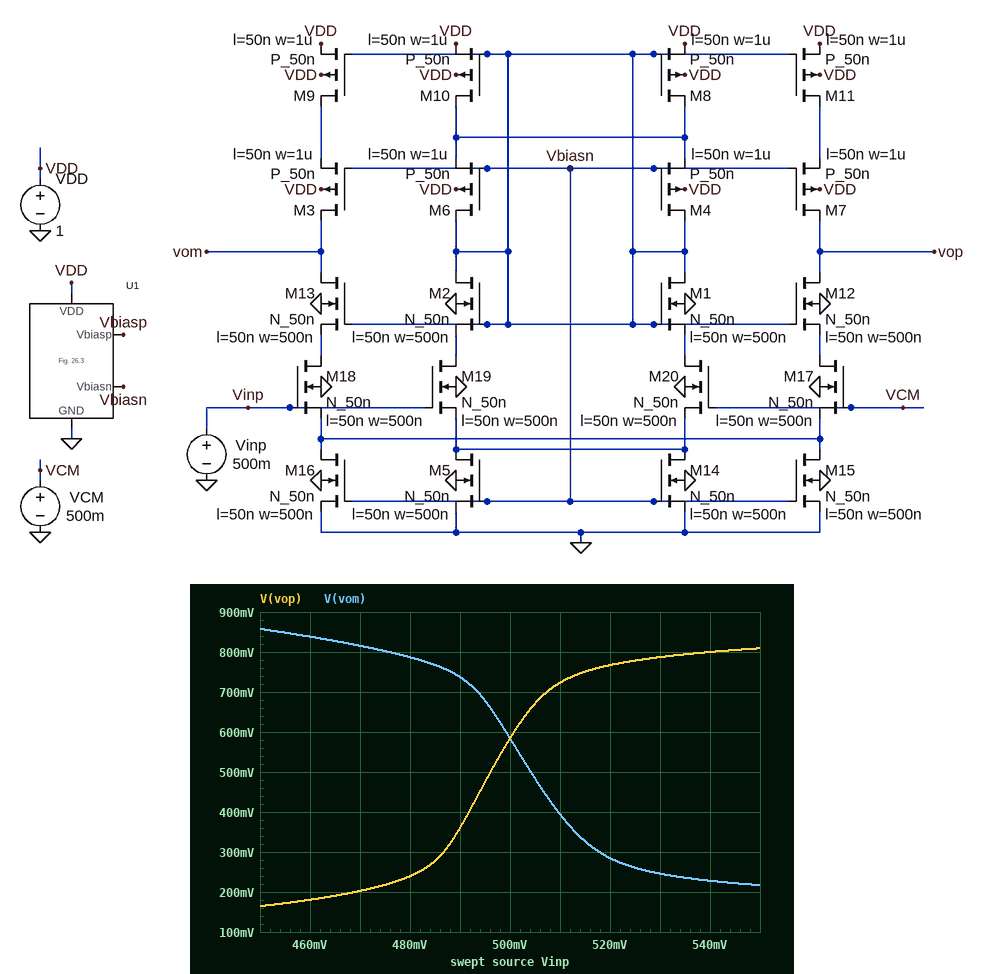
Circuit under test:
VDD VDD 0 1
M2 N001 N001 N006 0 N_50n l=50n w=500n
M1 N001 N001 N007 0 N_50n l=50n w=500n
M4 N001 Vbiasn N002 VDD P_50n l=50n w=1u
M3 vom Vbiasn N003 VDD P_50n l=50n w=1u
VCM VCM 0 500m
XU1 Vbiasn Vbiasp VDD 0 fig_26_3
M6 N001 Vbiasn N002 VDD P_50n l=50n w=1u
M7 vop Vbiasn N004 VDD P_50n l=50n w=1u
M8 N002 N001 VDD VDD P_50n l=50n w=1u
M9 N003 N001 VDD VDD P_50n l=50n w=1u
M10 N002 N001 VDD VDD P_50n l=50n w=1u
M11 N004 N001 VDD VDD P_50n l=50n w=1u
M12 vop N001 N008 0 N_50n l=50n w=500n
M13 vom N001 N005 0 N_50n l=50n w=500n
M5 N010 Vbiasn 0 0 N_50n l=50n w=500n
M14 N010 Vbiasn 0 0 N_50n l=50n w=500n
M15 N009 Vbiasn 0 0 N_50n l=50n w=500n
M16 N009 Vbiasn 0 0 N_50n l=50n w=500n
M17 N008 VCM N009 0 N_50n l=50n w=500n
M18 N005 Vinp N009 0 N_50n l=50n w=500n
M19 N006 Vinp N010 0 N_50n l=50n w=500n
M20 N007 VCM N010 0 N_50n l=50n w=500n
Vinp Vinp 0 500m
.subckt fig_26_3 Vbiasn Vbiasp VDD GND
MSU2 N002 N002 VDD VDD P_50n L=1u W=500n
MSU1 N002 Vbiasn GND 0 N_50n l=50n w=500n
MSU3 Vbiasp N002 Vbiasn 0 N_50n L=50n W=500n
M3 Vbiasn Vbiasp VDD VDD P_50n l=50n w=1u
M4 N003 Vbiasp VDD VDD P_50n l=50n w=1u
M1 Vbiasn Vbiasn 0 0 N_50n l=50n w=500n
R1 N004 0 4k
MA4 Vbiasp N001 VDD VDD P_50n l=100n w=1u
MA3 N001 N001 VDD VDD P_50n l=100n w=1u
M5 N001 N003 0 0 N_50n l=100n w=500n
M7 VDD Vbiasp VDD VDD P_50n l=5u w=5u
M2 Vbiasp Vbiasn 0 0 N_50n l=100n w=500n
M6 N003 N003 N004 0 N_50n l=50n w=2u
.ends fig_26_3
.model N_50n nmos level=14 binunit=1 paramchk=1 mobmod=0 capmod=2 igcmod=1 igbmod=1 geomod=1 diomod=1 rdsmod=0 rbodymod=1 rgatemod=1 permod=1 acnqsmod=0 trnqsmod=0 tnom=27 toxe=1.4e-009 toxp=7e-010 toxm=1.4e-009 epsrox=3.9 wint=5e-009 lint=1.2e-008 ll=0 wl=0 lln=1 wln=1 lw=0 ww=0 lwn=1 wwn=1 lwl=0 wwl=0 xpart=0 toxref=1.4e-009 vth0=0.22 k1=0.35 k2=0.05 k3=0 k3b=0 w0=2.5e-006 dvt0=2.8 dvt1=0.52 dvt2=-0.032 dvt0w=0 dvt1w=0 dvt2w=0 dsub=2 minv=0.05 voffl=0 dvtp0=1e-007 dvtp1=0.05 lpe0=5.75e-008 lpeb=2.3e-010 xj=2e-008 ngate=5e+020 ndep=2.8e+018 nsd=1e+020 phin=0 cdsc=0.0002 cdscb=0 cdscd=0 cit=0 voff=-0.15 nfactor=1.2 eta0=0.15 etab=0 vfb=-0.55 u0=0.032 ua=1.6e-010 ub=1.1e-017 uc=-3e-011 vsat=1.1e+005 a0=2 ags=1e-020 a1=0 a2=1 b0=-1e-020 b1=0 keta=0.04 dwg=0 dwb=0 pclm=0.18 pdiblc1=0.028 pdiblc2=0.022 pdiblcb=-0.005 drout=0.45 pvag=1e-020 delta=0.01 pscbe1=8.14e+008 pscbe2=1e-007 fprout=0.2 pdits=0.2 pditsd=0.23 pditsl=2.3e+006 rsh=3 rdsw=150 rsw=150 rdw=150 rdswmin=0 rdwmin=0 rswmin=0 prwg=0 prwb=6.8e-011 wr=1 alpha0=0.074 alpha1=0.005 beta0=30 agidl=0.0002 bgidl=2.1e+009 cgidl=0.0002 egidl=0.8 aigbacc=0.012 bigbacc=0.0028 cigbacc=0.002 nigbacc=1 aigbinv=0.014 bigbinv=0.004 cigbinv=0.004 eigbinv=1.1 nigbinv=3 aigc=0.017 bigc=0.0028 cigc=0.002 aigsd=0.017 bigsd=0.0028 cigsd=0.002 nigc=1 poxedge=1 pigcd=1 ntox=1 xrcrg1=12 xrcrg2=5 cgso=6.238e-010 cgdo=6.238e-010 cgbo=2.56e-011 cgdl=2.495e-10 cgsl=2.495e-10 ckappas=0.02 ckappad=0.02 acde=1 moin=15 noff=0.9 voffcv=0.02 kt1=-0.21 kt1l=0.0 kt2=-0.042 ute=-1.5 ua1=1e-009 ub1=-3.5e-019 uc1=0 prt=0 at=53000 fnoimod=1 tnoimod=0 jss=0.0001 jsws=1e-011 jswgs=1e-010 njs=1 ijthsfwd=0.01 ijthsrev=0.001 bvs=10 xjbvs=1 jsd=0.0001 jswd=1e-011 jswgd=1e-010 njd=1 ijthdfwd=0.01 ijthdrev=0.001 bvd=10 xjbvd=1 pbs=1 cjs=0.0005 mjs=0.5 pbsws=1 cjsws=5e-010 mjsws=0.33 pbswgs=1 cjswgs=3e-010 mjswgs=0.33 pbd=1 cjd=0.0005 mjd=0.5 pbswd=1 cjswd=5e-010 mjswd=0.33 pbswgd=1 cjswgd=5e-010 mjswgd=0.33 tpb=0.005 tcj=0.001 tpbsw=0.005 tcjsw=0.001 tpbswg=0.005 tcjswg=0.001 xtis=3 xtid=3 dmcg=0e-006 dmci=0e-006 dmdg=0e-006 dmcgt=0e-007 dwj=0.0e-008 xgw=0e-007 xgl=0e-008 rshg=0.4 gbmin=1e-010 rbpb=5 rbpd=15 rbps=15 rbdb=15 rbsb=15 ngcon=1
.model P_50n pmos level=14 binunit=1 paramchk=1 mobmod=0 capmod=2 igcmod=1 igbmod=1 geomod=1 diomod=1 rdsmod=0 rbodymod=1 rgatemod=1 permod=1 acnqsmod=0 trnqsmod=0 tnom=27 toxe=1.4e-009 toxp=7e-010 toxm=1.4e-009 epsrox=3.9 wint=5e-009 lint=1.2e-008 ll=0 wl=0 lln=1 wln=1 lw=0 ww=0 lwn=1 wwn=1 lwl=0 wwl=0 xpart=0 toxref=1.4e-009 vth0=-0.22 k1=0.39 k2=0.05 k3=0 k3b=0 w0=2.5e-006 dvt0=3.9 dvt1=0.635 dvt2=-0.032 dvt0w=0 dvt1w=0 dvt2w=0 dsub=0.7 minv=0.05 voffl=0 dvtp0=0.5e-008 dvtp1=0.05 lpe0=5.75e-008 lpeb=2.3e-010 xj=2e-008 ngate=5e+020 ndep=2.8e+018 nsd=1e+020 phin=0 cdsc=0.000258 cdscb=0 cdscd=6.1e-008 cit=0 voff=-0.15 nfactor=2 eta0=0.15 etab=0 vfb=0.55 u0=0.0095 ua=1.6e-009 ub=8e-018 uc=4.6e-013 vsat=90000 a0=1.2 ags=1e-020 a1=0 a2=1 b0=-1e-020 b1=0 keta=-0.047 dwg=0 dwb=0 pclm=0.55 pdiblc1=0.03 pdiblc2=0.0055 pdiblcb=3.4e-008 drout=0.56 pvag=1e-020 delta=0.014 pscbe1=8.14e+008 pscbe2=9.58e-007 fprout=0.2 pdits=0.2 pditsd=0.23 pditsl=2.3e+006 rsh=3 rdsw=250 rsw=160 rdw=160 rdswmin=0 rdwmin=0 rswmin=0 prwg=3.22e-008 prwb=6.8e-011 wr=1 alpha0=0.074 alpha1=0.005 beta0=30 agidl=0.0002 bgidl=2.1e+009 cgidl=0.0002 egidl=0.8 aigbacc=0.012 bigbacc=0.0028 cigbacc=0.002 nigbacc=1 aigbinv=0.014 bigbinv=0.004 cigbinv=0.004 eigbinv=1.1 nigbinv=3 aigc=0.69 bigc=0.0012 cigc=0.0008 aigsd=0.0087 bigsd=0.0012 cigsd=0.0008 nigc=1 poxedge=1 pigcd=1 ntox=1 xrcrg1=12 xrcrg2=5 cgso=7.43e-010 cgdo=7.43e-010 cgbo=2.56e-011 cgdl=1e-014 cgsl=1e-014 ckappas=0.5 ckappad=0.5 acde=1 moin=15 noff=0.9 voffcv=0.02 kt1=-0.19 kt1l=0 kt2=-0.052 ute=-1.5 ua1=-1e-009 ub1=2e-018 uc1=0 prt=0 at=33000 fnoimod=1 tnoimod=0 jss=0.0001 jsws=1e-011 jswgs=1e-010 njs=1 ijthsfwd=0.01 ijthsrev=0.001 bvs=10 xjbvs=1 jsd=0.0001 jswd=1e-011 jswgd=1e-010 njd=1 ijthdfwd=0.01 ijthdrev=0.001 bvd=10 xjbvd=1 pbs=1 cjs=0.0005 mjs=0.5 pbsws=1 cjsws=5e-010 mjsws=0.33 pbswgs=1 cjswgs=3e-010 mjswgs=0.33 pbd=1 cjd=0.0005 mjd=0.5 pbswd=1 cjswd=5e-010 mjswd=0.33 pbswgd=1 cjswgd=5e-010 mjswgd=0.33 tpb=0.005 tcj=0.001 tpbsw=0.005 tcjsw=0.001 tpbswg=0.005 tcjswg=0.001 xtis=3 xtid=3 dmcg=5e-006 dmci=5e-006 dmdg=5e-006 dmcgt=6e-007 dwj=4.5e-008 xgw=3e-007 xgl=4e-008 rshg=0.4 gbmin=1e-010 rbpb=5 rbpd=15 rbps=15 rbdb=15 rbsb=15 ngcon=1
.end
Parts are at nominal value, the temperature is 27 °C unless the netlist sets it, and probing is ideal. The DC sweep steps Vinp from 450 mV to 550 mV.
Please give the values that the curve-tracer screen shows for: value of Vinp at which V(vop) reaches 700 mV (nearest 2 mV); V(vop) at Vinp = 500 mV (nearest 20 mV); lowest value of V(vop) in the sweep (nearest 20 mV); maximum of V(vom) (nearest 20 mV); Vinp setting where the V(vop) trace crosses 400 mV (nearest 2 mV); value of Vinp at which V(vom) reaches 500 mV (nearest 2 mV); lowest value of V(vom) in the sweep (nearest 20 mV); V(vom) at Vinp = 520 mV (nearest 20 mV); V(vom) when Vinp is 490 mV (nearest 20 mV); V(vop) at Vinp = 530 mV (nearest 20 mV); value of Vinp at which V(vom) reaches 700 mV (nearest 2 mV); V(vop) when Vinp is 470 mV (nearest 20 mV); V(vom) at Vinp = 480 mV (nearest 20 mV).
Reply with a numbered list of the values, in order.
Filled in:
1. 508 mV
2. 580 mV
3. 160 mV
4. 860 mV
5. 492 mV
6. 504 mV
7. 220 mV
8. 280 mV
9. 740 mV
10. 780 mV
11. 494 mV
12. 200 mV
13. 780 mV
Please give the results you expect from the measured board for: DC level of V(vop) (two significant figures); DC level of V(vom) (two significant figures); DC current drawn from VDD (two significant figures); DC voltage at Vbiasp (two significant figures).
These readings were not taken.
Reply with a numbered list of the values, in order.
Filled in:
1. 580 mV
2. 580 mV
3. 110 µA
4. 590 mV
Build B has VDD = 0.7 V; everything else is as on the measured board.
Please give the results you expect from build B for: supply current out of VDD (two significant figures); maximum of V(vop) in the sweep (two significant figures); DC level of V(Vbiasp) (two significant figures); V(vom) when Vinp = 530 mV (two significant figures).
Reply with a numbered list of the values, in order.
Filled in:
1. 58 µA
2. 300 mV
3. 270 mV
4. 290 mV
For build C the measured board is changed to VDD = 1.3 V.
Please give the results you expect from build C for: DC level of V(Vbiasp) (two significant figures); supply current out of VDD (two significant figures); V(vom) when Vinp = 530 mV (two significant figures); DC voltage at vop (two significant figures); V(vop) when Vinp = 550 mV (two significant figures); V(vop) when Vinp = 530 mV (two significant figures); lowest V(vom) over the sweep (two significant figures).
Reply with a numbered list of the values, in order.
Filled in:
1. 910 mV
2. 120 µA
3. 320 mV
4. 900 mV
5. 1.1 V
6. 1.0 V
7. 230 mV
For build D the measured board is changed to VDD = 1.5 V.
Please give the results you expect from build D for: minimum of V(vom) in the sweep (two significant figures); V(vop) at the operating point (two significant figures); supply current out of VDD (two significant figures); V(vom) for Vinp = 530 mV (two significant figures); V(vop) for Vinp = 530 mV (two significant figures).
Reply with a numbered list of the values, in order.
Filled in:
1. 490 mV
2. 1.1 V
3. 130 µA
4. 860 mV
5. 1.3 V
